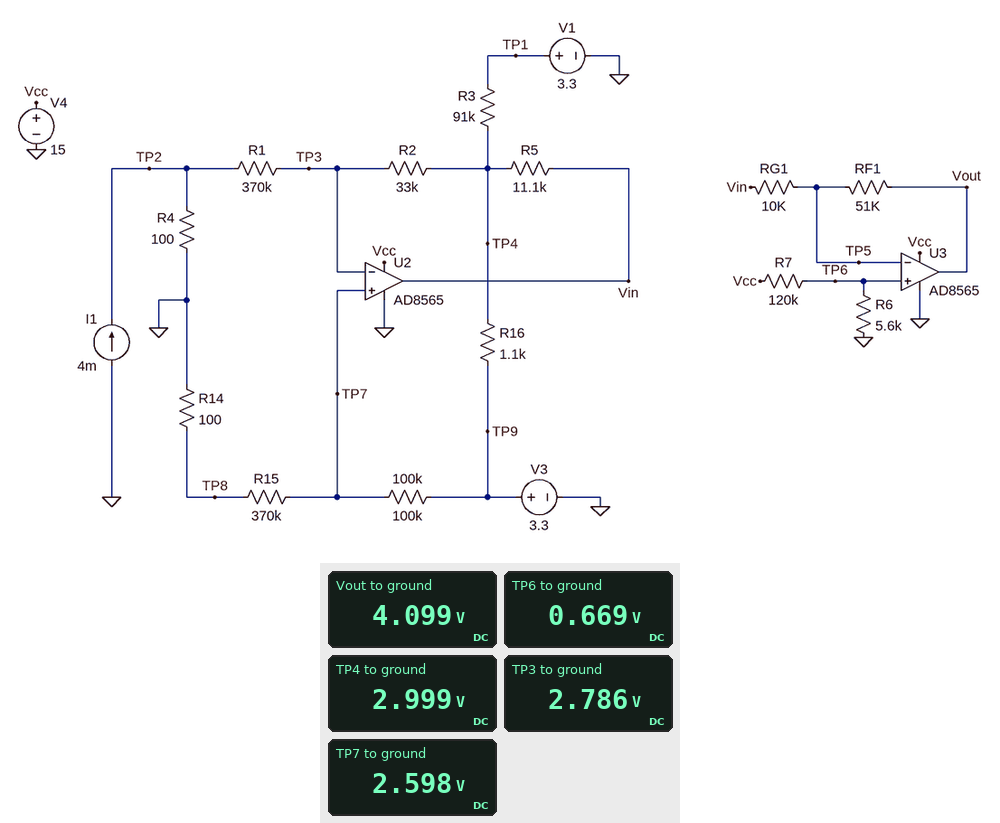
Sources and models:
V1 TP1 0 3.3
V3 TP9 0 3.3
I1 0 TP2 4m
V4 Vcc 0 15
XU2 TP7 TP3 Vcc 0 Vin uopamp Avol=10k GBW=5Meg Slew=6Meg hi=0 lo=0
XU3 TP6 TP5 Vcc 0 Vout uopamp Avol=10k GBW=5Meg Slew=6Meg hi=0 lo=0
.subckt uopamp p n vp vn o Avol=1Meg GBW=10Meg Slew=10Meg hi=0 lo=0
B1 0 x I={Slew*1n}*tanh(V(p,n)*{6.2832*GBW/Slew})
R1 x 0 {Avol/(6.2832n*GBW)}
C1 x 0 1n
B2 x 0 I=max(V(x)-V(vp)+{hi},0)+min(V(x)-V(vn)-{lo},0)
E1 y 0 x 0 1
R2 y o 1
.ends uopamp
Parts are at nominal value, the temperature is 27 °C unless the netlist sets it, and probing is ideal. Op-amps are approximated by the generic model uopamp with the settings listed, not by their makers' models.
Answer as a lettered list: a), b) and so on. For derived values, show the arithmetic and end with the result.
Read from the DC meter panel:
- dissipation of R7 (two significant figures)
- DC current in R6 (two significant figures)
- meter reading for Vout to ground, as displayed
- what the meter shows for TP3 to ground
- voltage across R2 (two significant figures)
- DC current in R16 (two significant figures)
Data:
a) (15 V - 669 mV)^2 / 120 kΩ = 1.7 mW
b) (669 mV) / 5.6 kΩ = 120 µA
c) 4.099 V
d) 2.786 V
e) 2.999 V - 2.786 V = 210 mV
f) (3.3 V - 2.999 V) / 1.1 kΩ = 270 µA
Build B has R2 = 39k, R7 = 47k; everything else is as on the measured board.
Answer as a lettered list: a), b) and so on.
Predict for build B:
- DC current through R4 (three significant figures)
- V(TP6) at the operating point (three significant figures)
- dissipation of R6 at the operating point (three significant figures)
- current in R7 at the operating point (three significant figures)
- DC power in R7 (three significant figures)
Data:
a) 4.01 mA
b) 1.60 V
c) 455 µW
d) 285 µA
e) 3.82 mW
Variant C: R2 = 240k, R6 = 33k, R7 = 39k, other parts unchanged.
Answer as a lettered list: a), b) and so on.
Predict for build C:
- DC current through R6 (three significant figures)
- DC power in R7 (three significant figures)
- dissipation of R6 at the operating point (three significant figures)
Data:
a) 208 µA
b) 1.69 mW
c) 1.43 mW
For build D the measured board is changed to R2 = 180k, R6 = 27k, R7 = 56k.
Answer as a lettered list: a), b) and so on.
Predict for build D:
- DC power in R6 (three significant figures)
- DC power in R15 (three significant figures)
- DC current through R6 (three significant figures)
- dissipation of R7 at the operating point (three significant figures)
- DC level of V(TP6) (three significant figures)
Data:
a) 882 µW
b) 18.2 µW
c) 181 µA
d) 1.83 mW
e) 4.88 V
